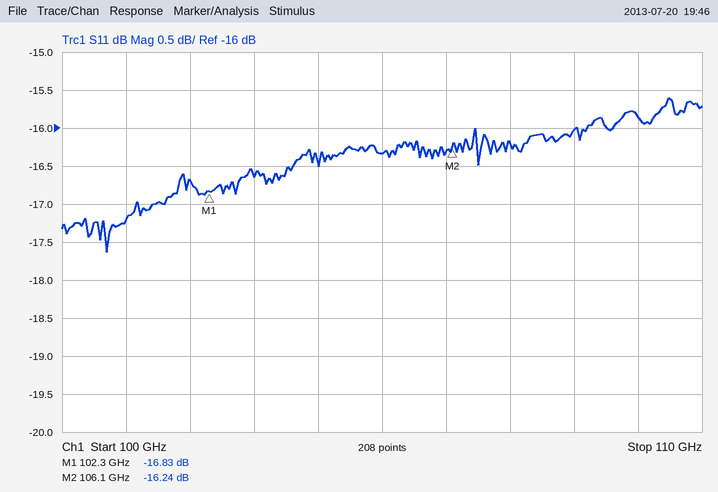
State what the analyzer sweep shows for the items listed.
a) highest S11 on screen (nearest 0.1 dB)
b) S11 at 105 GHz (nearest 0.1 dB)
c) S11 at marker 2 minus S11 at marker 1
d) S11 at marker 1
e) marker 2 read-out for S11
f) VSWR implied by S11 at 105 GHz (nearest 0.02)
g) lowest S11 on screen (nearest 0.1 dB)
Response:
-15.6 dB
-16.3 dB
0.59 dB
-16.83 dB
-16.24 dB
1.36
-17.6 dB
